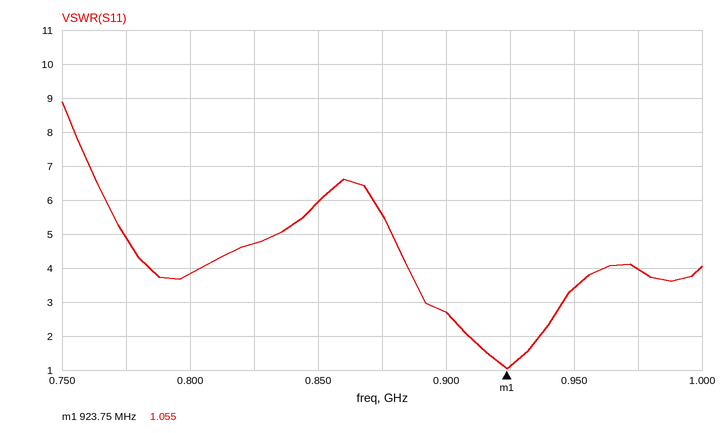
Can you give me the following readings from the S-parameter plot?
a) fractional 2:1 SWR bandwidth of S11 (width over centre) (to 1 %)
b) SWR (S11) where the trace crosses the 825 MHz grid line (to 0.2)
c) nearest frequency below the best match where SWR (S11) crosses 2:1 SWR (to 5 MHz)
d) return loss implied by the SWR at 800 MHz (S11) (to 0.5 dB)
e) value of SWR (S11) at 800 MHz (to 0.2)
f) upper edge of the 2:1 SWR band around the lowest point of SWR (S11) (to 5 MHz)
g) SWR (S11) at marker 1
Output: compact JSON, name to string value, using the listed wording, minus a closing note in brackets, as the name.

{"fractional 2:1 SWR bandwidth of S11 (width over centre)": "3 %", "SWR (S11) where the trace crosses the 825 MHz grid line": "4.8", "nearest frequency below the best match where SWR (S11) crosses 2:1 SWR": "910 MHz", "return loss implied by the SWR at 800 MHz (S11)": "4.5 dB", "value of SWR (S11) at 800 MHz": "3.8", "upper edge of the 2:1 SWR band around the lowest point of SWR (S11)": "935 MHz", "SWR (S11) at marker 1": "1.055"}
